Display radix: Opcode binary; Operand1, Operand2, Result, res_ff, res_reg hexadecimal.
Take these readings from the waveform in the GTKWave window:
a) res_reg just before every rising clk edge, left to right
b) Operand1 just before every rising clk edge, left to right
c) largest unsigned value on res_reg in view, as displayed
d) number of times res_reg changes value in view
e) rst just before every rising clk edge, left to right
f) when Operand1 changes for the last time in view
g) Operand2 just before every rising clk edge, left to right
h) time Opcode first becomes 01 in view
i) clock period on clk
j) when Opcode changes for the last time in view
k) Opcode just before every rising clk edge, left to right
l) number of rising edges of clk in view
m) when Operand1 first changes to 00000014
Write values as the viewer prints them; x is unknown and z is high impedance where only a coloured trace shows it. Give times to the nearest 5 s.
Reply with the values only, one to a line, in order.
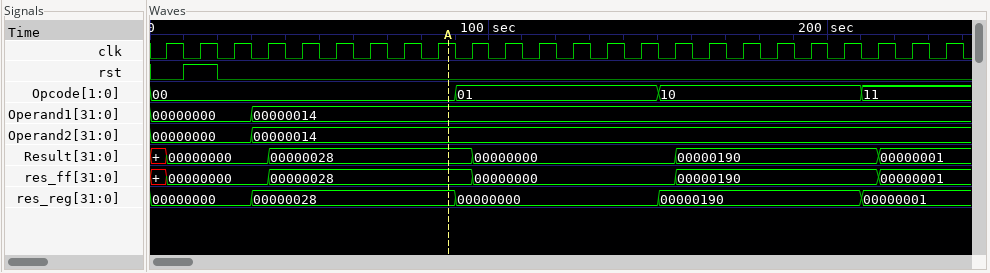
00000000, 00000000, 00000000, 00000028, 00000028, 00000028, 00000028, 00000028, 00000028, 00000000, 00000000, 00000000, 00000000, 00000000, 00000000, 00000190, 00000190, 00000190, 00000190, 00000190, 00000190, 00000001, 00000001, 00000001
00000000, 00000000, 00000000, 00000014, 00000014, 00000014, 00000014, 00000014, 00000014, 00000014, 00000014, 00000014, 00000014, 00000014, 00000014, 00000014, 00000014, 00000014, 00000014, 00000014, 00000014, 00000014, 00000014, 00000014
00000190
4
0 1 0 0 0 0 0 0 0 0 0 0 0 0 0 0 0 0 0 0 0 0 0 0
30 s
00000000, 00000000, 00000000, 00000014, 00000014, 00000014, 00000014, 00000014, 00000014, 00000014, 00000014, 00000014, 00000014, 00000014, 00000014, 00000014, 00000014, 00000014, 00000014, 00000014, 00000014, 00000014, 00000014, 00000014
90 s
10 s
210 s
00, 00, 00, 00, 00, 00, 00, 00, 00, 01, 01, 01, 01, 01, 01, 10, 10, 10, 10, 10, 10, 11, 11, 11
24
30 s
